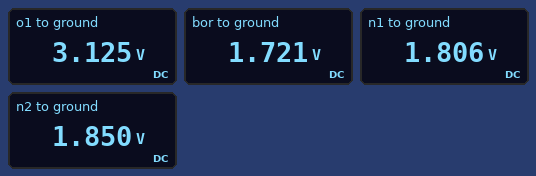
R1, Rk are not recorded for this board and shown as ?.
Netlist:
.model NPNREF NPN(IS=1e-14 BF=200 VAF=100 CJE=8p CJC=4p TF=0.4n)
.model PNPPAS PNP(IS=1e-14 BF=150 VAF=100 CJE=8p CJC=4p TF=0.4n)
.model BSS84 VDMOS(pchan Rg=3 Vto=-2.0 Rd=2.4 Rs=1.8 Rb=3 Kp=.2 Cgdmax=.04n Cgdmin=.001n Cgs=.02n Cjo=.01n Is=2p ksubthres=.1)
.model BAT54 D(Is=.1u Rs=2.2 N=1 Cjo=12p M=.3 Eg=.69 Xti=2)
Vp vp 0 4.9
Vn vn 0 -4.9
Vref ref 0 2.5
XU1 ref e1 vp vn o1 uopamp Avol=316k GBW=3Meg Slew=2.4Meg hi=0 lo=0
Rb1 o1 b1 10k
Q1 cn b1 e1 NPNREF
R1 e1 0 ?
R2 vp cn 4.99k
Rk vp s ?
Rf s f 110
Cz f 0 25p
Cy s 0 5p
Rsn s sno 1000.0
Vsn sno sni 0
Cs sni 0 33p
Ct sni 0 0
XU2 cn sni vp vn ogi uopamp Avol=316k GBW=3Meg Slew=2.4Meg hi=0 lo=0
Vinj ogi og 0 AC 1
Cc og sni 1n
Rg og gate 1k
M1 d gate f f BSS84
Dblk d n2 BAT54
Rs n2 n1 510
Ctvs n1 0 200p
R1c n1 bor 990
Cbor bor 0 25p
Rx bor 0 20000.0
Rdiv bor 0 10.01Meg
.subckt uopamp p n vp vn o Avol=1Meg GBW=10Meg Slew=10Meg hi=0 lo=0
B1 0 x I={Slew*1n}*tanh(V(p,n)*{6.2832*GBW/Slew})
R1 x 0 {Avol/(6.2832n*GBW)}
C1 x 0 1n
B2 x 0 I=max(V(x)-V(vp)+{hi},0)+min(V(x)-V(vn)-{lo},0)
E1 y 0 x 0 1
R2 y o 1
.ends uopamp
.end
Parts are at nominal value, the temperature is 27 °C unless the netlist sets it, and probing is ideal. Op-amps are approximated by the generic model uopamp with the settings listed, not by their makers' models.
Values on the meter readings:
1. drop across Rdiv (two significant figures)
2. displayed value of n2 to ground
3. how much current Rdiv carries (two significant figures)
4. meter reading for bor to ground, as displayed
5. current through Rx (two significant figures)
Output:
1.7 V
1.850 V
170 nA
1.721 V
86 µA
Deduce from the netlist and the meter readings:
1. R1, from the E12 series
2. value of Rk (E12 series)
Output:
12 kΩ
12 kΩ
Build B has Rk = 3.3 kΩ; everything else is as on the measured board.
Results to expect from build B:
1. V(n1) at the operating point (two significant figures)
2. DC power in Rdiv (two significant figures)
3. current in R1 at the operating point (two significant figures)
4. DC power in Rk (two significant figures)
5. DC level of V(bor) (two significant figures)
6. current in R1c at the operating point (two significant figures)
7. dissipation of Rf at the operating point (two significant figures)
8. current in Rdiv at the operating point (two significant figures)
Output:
4.0 V
1.4 µW
210 µA
120 µW
3.8 V
190 µA
3.9 µW
380 nA
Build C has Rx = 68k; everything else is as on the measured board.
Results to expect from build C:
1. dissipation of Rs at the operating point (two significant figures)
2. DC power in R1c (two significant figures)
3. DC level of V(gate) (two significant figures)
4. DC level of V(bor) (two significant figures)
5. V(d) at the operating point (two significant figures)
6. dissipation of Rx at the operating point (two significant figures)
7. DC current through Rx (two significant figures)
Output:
1.7 µW
3.4 µW
-4.9 V
3.9 V
4.2 V
230 µW
58 µA
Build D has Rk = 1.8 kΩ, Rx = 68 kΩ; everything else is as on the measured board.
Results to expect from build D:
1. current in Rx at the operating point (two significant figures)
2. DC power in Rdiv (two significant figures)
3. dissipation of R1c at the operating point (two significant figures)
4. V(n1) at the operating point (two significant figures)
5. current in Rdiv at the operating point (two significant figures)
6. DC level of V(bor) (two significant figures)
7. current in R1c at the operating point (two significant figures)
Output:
66 µA
2.0 µW
4.4 µW
4.6 V
450 nA
4.5 V
67 µA
